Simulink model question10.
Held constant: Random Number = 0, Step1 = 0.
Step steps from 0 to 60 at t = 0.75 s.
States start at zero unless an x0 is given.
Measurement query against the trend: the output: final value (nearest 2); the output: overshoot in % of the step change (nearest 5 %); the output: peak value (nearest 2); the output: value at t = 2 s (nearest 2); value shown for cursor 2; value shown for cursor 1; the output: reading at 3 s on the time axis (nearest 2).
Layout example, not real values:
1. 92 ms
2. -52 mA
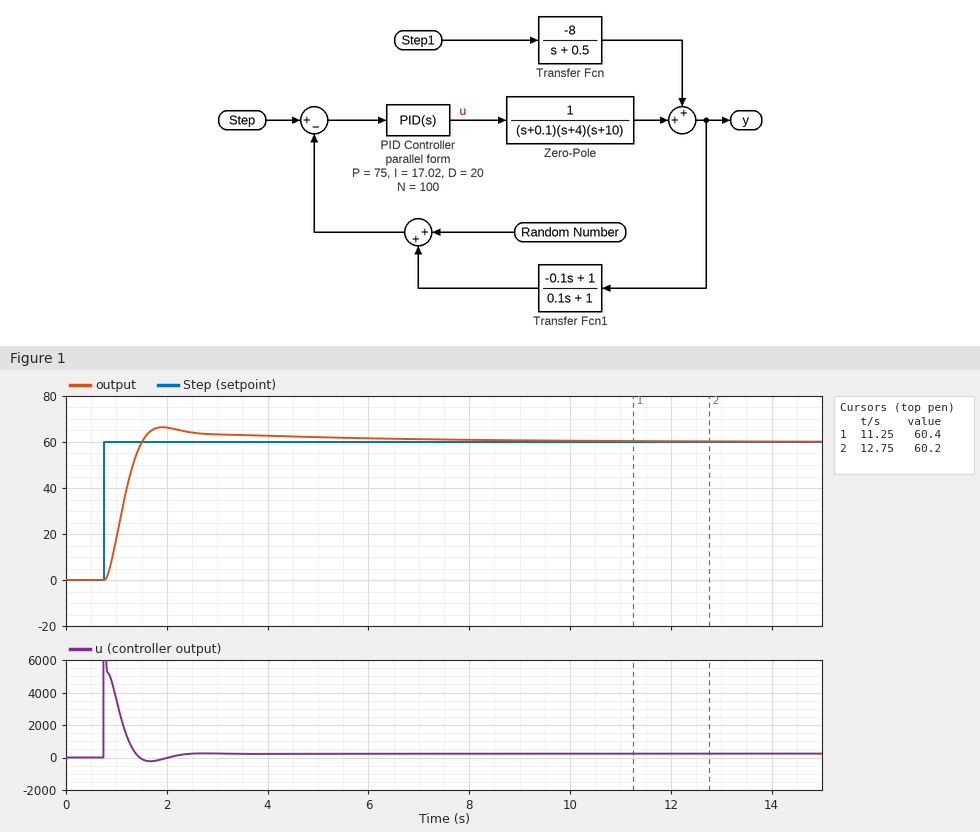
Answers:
1. 60
2. 10 %
3. 66
4. 66
5. 60.2
6. 60.4
7. 64
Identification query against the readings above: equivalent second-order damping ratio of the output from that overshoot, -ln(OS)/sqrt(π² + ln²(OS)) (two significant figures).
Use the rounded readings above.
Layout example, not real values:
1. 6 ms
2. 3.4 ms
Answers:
1. 0.59
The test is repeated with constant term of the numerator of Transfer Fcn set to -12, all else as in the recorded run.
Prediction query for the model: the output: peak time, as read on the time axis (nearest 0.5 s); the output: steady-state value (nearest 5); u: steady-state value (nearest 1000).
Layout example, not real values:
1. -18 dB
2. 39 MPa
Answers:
1. 2.0 s
2. 60
3. 0
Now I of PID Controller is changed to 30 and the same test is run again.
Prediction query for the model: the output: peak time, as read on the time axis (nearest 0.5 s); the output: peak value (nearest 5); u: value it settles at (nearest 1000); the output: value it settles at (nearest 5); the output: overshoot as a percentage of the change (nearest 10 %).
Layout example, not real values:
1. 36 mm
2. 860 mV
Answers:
1. 2.0 s
2. 70
3. 0
4. 60
5. 20 %
